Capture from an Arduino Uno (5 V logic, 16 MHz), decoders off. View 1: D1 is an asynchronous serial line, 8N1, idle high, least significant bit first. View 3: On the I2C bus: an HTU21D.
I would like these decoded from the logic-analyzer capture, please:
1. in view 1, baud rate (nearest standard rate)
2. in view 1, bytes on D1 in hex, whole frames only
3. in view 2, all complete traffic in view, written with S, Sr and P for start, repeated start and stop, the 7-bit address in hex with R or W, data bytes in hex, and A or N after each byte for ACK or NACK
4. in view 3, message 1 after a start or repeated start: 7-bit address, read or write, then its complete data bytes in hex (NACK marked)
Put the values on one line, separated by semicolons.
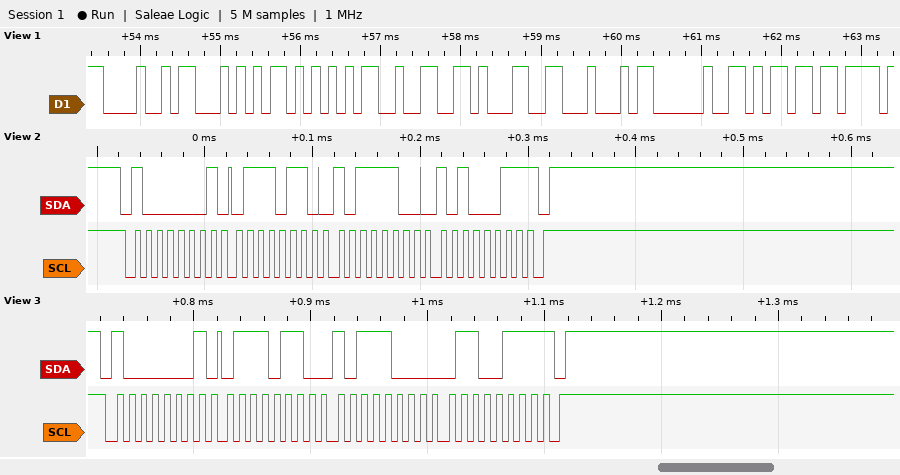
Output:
9600 baud; 0x48 0x54 0x55 0x32 0x31 0x44 0x20 0x6D; S 40R A 76 A BC A A3 N P; 0x40 read: 76 B8 67 NACK
